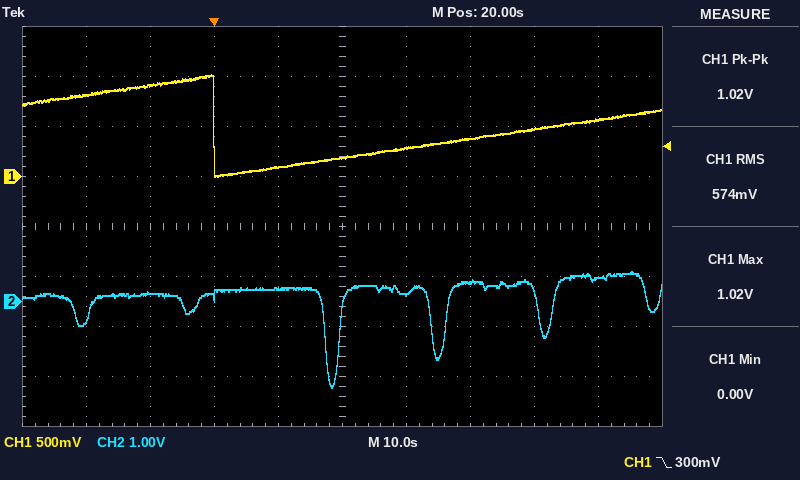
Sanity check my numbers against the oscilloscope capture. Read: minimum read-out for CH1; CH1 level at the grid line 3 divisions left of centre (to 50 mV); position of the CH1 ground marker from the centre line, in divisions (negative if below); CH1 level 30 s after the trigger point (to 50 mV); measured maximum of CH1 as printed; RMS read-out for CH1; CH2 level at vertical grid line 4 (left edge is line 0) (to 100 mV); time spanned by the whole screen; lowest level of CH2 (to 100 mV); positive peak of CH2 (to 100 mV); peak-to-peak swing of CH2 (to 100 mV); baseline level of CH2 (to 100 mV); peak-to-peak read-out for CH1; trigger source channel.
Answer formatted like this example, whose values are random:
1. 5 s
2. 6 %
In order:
1. 0.00 V
2. 900 mV
3. +1.0 div
4. 300 mV
5. 1.02 V
6. 574 mV
7. 300 mV
8. 100 s
9. -1.7 V
10. 600 mV
11. 2.3 V
12. 200 mV
13. 1.02 V
14. CH1
